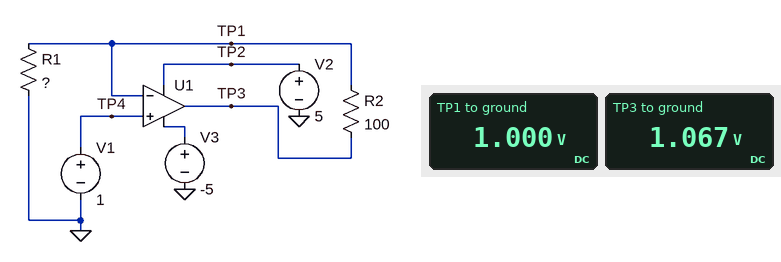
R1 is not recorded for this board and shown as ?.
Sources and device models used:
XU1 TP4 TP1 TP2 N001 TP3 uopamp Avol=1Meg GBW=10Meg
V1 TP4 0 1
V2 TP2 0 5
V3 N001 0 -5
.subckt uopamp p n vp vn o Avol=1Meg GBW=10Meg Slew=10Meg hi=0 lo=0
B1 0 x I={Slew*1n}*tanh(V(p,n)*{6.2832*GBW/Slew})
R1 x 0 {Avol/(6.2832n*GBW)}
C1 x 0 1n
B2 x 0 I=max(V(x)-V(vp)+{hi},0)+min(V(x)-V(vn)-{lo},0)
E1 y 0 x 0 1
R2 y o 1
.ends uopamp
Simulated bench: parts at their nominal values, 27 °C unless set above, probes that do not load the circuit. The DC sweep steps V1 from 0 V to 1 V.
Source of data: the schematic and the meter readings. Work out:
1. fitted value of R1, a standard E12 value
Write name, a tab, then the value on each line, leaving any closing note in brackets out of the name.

fitted value of R1, a standard E12 value	1.5 kΩ
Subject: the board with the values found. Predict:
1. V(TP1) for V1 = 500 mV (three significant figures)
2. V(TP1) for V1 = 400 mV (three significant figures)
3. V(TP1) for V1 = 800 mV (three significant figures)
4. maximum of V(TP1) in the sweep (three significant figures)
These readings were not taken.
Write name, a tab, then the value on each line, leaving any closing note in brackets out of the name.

V(TP1) for V1 = 500 mV	500 mV
V(TP1) for V1 = 400 mV	400 mV
V(TP1) for V1 = 800 mV	800 mV
maximum of V(TP1) in the sweep	1.00 V
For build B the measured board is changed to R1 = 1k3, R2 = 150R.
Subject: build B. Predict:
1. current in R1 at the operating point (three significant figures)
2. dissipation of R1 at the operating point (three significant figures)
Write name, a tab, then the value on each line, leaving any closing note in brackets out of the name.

current in R1 at the operating point	769 µA
dissipation of R1 at the operating point	769 µW
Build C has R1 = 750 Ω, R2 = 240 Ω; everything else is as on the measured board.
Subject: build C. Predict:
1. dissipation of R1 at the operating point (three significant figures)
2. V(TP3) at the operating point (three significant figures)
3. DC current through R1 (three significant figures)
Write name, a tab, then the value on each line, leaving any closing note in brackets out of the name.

dissipation of R1 at the operating point	1.33 mW
V(TP3) at the operating point	1.32 V
DC current through R1	1.33 mA
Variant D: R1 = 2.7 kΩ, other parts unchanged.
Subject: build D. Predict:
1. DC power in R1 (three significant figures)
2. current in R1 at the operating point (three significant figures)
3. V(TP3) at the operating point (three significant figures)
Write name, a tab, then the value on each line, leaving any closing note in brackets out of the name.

DC power in R1	370 µW
current in R1 at the operating point	370 µA
V(TP3) at the operating point	1.04 V
